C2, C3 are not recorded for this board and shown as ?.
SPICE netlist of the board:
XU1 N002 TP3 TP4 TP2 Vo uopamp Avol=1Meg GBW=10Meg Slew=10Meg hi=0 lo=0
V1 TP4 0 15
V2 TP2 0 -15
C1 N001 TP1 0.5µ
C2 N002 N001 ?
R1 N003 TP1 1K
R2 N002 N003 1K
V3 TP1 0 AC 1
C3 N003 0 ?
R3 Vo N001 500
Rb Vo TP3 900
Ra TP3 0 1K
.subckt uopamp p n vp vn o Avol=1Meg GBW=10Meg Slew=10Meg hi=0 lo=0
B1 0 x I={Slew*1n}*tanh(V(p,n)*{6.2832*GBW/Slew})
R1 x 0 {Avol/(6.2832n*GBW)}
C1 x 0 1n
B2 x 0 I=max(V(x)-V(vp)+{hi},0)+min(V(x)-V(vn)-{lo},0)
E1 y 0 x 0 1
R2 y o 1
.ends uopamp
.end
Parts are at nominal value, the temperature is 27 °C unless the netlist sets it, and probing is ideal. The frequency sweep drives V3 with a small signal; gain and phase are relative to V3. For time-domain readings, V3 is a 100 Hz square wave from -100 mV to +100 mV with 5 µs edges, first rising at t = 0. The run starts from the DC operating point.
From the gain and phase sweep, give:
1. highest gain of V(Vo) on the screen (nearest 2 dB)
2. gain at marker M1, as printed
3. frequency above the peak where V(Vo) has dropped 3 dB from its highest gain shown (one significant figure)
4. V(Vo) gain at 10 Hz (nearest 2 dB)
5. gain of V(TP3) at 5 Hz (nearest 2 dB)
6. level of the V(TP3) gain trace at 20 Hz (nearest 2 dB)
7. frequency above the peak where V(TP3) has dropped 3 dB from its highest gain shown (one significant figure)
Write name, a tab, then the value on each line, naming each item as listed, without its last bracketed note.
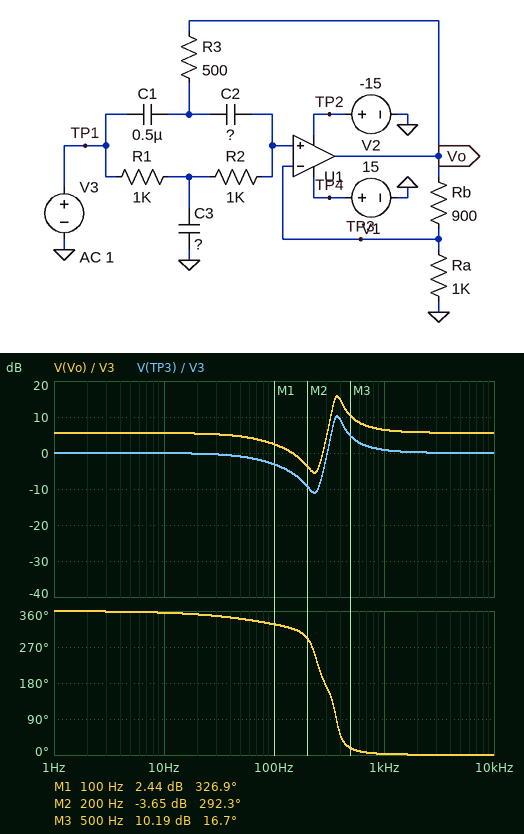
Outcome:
highest gain of V(Vo) on the screen	16 dB
gain at marker M1, as printed	2.44 dB
frequency above the peak where V(Vo) has dropped 3 dB from its highest gain shown	400 Hz
V(Vo) gain at 10 Hz	6 dB
gain of V(TP3) at 5 Hz	0 dB
level of the V(TP3) gain trace at 20 Hz	0 dB
frequency above the peak where V(TP3) has dropped 3 dB from its highest gain shown	400 Hz
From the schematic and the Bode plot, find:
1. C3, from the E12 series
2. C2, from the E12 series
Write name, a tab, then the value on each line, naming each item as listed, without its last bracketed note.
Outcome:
C3, from the E12 series	2.2 µF
C2, from the E12 series	560 nF
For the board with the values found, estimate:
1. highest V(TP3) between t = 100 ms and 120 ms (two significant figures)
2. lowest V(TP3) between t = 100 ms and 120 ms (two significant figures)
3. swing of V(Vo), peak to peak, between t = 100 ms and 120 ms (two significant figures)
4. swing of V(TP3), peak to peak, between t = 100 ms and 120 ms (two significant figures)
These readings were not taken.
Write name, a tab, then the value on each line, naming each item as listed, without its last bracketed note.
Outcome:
highest V(TP3) between t = 100 ms and 120 ms	140 mV
lowest V(TP3) between t = 100 ms and 120 ms	-140 mV
swing of V(Vo), peak to peak, between t = 100 ms and 120 ms	530 mV
swing of V(TP3), peak to peak, between t = 100 ms and 120 ms	280 mV
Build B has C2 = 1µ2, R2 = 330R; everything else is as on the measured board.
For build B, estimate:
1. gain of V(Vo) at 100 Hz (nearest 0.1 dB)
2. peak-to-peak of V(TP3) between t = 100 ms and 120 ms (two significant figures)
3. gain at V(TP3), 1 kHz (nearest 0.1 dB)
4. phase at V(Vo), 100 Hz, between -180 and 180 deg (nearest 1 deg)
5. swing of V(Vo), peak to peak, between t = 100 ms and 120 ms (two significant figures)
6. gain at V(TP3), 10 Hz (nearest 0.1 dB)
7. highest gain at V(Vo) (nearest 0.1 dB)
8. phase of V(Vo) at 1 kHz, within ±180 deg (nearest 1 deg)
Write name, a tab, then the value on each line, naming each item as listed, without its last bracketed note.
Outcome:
gain of V(Vo) at 100 Hz	4.9 dB
peak-to-peak of V(TP3) between t = 100 ms and 120 ms	230 mV
gain at V(TP3), 1 kHz	-3.1 dB
phase at V(Vo), 100 Hz, between -180 and 180 deg	-37 deg
swing of V(Vo), peak to peak, between t = 100 ms and 120 ms	440 mV
gain at V(TP3), 10 Hz	0 dB
highest gain at V(Vo)	5.6 dB
phase of V(Vo) at 1 kHz, within ±180 deg	36 deg
